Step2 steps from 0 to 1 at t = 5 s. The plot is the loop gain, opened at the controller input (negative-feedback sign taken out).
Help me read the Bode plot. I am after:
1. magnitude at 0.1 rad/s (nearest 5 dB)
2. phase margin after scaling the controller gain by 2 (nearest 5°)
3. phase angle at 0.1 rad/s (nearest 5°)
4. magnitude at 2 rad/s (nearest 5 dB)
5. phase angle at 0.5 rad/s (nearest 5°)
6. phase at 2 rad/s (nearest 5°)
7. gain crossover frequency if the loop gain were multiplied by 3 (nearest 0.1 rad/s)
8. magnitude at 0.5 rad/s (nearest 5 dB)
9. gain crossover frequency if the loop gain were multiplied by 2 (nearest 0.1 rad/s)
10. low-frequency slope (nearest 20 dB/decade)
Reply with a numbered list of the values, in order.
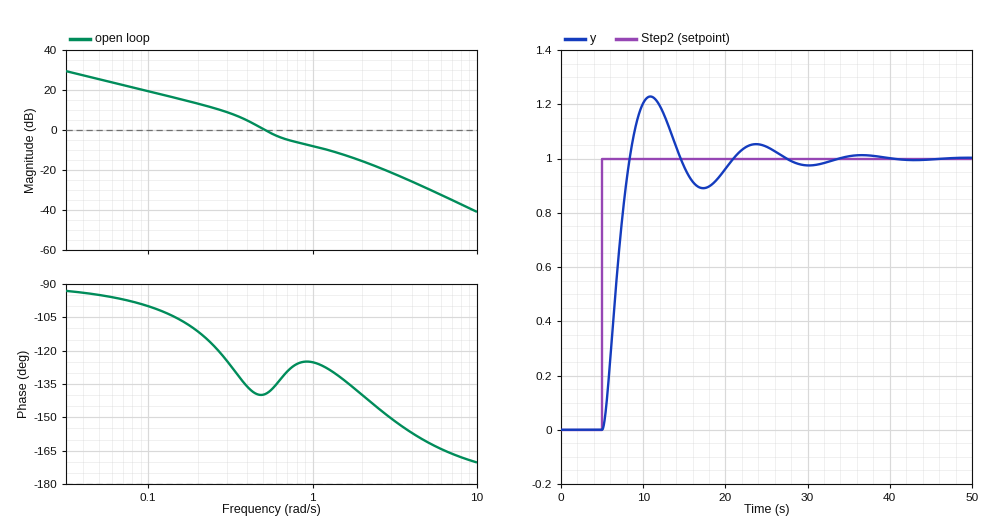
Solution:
1. 20 dB
2. 55°
3. -100°
4. -15 dB
5. -140°
6. -140°
7. 1.2 rad/s
8. 0 dB
9. 0.8 rad/s
10. -20 dB/decade
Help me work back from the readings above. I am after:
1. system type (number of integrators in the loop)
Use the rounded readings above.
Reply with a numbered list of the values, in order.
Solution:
1. 1
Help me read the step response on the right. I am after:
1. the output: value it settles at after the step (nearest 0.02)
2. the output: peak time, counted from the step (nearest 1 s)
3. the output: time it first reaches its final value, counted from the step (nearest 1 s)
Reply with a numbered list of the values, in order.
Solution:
1. 1.00
2. 6 s
3. 3 s
